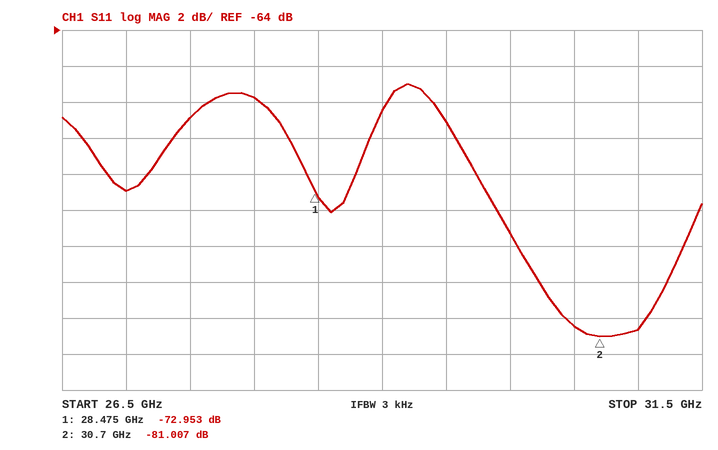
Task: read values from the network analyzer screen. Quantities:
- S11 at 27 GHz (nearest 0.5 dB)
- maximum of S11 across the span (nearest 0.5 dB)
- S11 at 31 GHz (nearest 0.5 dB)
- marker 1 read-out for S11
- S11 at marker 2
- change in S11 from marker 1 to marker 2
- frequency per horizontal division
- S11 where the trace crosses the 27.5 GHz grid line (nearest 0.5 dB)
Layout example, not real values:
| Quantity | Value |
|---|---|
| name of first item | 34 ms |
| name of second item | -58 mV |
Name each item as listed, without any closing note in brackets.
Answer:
| Quantity | Value |
|---|---|
| S11 at 27 GHz | -73.0 dB |
| maximum of S11 across the span | -67.0 dB |
| S11 at 31 GHz | -80.5 dB |
| marker 1 read-out for S11 | -72.953 dB |
| S11 at marker 2 | -81.007 dB |
| change in S11 from marker 1 to marker 2 | -8.054 dB |
| frequency per horizontal division | 500 MHz |
| S11 where the trace crosses the 27.5 GHz grid line | -69.0 dB |
